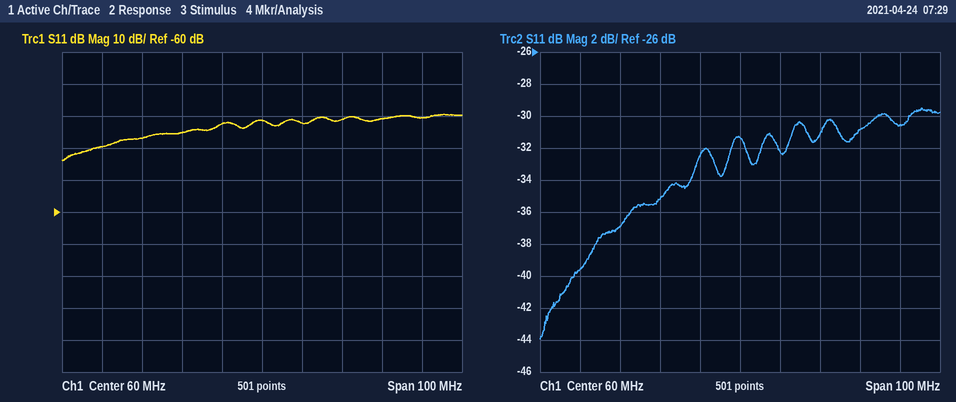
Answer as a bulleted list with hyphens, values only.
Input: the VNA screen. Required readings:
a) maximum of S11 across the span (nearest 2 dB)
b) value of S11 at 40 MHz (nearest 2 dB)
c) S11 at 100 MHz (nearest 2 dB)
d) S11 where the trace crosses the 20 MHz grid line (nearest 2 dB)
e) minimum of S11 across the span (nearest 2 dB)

- -30 dB
- -36 dB
- -30 dB
- -40 dB
- -44 dB
